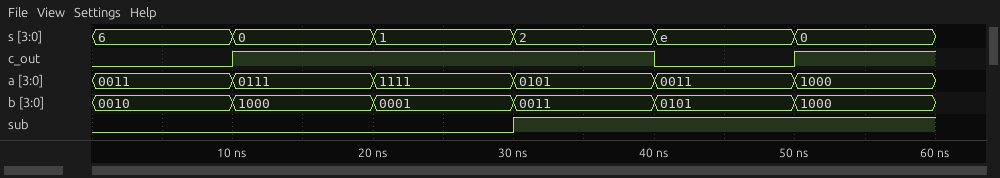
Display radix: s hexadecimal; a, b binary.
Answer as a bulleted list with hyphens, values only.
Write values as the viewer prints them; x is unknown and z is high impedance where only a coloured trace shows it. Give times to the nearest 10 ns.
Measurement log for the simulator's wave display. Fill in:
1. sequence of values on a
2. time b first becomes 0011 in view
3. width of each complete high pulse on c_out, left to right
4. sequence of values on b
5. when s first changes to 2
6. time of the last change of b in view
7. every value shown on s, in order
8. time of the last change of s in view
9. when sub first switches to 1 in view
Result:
- 0011, 0111, 1111, 0101, 0011, 1000
- 30 ns
- 30 ns
- 0010, 1000, 0001, 0011, 0101, 1000
- 30 ns
- 50 ns
- 6, 0, 1, 2, e, 0
- 50 ns
- 30 ns
